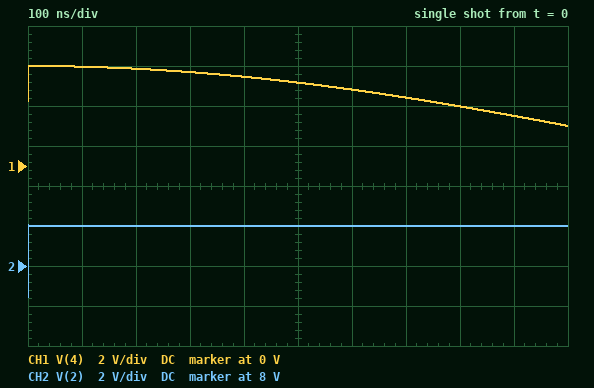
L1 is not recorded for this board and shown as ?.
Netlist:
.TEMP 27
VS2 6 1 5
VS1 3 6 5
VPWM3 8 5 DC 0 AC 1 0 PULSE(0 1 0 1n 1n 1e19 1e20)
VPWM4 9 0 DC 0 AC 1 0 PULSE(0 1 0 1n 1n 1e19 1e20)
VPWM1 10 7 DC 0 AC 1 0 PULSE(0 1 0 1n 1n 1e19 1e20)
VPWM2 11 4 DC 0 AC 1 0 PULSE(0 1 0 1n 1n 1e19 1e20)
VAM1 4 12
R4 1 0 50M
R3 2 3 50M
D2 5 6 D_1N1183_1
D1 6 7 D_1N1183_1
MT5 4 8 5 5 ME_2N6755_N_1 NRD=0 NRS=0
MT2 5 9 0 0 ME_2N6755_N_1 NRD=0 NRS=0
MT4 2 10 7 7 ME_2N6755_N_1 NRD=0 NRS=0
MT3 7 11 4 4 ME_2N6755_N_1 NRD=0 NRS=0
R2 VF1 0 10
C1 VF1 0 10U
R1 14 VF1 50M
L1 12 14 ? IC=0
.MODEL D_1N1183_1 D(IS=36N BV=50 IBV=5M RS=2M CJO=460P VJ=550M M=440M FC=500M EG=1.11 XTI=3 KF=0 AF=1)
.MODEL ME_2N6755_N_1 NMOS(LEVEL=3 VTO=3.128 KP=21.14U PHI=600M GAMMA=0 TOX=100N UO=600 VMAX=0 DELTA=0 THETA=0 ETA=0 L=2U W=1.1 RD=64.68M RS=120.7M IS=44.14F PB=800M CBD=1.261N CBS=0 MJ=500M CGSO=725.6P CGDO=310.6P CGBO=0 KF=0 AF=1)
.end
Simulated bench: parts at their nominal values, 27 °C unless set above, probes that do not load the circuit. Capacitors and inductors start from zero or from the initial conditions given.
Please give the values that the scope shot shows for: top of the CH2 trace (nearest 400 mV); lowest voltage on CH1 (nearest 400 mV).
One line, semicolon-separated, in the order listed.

10.0 V; 2.0 V
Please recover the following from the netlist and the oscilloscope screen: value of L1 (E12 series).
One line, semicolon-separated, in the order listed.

680 µH
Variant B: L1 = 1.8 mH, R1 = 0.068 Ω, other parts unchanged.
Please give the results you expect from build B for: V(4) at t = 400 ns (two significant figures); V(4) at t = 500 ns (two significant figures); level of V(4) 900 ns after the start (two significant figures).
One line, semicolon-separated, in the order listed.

4.8 V; 4.7 V; 4.0 V
